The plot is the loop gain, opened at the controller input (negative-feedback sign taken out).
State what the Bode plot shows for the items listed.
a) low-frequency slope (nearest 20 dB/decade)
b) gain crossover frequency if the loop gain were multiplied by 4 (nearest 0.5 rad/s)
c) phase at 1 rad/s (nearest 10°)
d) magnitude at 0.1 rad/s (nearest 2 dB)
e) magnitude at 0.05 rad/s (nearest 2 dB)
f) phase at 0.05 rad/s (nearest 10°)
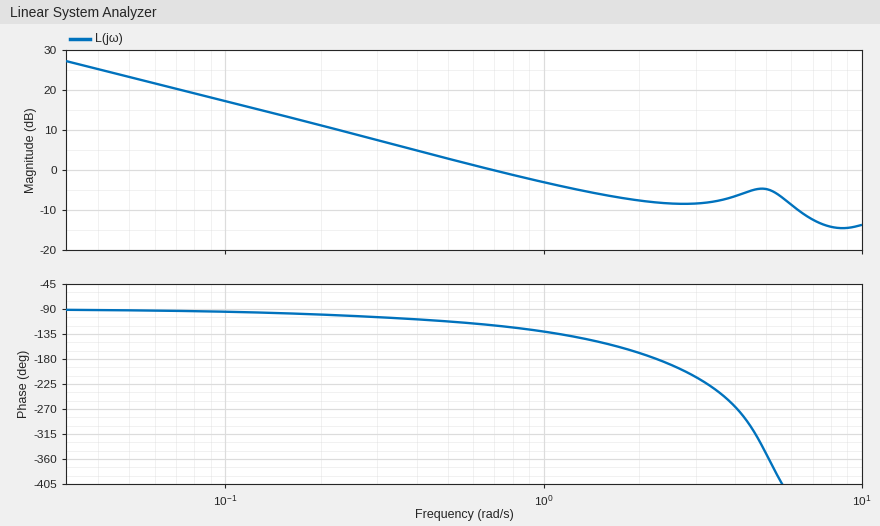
-20 dB/decade
7.0 rad/s
-130°
18 dB
24 dB
-90°
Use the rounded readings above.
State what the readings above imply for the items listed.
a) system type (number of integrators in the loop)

1
